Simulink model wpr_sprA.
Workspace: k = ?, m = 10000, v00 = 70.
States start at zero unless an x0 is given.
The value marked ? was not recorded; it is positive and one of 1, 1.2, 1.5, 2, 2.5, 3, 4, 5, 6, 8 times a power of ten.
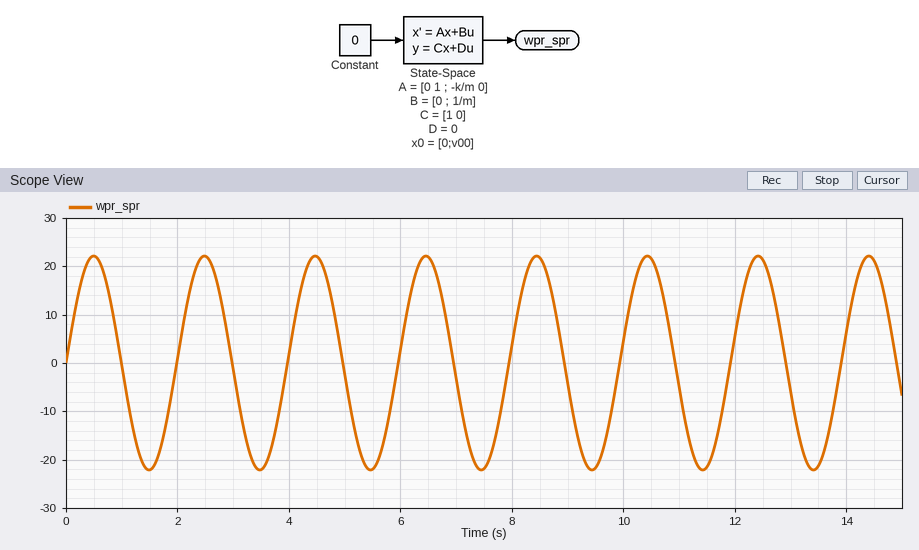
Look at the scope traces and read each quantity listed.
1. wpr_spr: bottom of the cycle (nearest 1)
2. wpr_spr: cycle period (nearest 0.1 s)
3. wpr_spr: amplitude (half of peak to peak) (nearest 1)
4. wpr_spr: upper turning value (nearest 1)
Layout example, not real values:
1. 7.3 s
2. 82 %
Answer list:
1. -22
2. 2.0 s
3. 22
4. 22
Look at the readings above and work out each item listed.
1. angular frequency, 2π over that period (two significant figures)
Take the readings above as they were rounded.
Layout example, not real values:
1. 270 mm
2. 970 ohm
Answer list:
1. 3.1 rad/s
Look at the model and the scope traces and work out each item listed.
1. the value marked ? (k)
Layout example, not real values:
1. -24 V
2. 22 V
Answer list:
1. 100000
